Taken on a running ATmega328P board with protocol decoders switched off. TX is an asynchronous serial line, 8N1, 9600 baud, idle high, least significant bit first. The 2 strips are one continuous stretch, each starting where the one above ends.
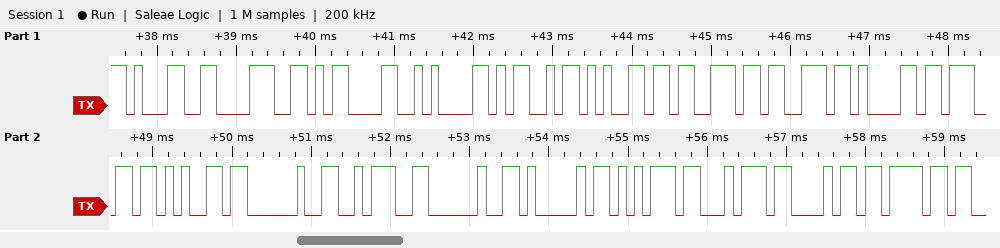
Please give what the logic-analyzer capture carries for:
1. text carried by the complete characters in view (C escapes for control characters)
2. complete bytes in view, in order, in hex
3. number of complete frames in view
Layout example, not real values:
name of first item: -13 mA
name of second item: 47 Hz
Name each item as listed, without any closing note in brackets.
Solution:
text carried by the complete characters in view: "18\r\nMessage : Autho"
complete bytes in view, in order, in hex: 31 38 0D 0A 4D 65 73 73 61 67 65 20 3A 20 41 75 74 68 6F
number of complete frames in view: 19
